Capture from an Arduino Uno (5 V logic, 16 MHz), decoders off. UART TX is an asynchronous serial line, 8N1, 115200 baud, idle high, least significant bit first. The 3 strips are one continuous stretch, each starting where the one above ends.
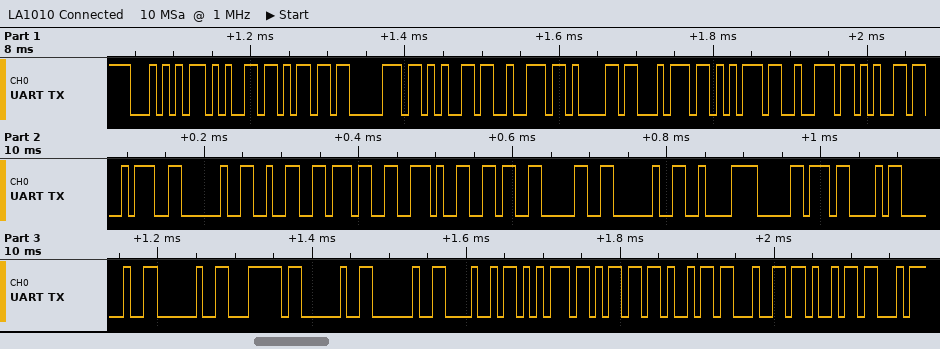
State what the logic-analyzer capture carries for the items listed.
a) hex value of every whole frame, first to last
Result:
54 65 6D 70 65 72 61 74 75 72 65 3A 20 32 37 2E 36 30 20 C2 B0 43 20 20 7C 20 20 48 75 6D 69 64 69
